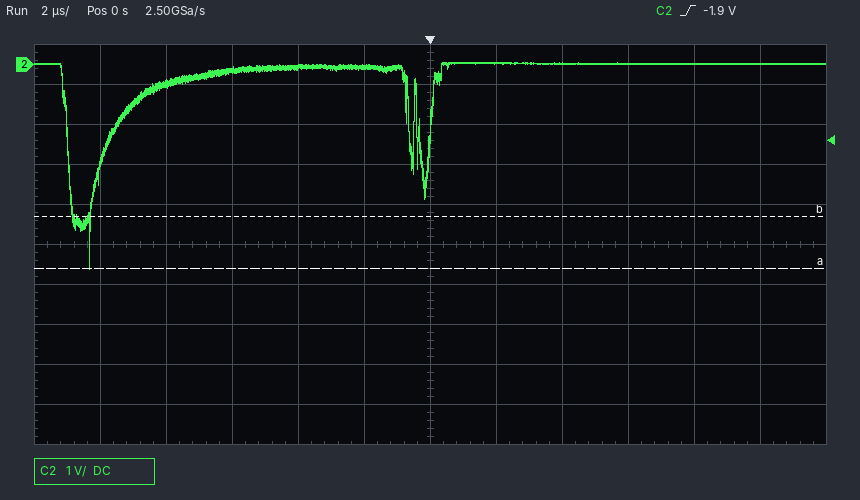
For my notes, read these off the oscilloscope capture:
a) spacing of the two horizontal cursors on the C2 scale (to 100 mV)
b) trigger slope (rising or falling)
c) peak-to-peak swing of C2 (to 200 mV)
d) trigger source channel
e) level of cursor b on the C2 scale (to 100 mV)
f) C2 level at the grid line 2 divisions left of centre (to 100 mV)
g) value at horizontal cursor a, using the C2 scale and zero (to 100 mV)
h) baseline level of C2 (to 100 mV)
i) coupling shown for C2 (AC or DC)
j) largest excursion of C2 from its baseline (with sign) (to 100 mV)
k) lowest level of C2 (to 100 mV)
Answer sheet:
1.3 V
rising
5.2 V
C2
-3.8 V
-100 mV
-5.1 V
0.0 V
DC
-5.1 V
-5.1 V
